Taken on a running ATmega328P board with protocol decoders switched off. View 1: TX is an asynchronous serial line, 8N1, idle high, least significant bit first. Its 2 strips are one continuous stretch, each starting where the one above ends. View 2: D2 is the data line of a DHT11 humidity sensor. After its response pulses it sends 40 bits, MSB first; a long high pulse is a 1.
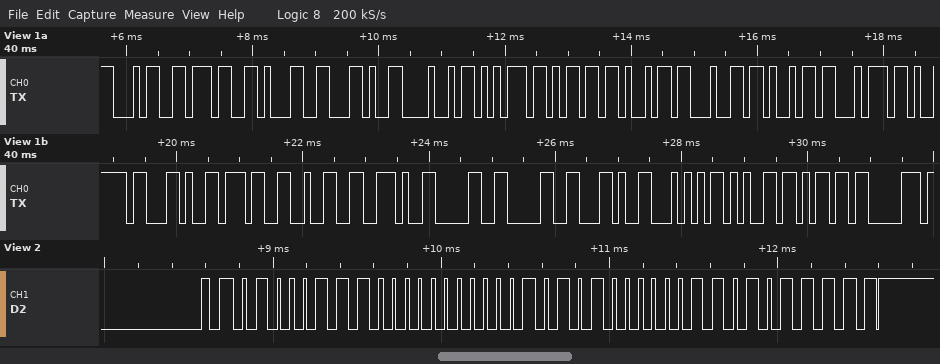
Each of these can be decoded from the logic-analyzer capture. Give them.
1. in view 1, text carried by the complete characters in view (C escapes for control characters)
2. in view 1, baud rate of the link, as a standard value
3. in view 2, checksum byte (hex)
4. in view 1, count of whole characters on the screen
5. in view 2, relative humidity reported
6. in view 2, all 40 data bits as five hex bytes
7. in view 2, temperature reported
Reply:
"471,Humidity,72.00,Temp"
9600 baud
0x5F
23
71 %
47 00 15 03 5F
21.3 °C
